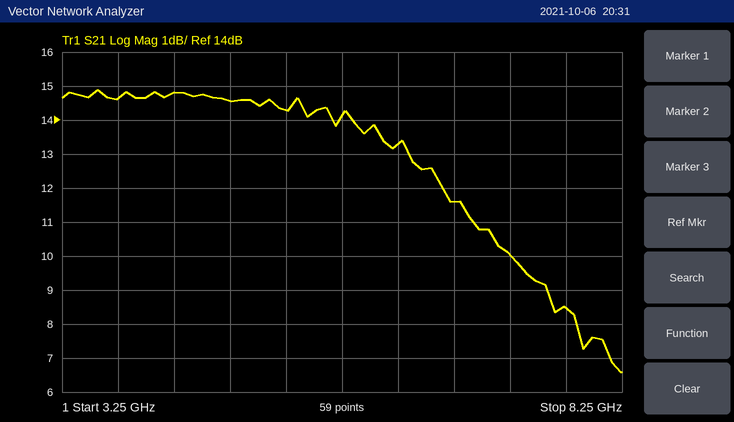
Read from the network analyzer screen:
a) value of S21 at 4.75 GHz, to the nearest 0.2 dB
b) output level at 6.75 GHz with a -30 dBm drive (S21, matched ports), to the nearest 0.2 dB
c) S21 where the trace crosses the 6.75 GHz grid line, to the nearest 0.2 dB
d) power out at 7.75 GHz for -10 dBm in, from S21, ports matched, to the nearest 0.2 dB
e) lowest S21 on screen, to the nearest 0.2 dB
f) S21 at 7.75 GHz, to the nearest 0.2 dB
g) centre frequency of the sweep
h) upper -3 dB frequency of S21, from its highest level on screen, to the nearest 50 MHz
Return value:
14.6 dB
-18.4 dBm
11.6 dB
-1.6 dBm
6.6 dB
8.4 dB
5.75 GHz
6.65 GHz
